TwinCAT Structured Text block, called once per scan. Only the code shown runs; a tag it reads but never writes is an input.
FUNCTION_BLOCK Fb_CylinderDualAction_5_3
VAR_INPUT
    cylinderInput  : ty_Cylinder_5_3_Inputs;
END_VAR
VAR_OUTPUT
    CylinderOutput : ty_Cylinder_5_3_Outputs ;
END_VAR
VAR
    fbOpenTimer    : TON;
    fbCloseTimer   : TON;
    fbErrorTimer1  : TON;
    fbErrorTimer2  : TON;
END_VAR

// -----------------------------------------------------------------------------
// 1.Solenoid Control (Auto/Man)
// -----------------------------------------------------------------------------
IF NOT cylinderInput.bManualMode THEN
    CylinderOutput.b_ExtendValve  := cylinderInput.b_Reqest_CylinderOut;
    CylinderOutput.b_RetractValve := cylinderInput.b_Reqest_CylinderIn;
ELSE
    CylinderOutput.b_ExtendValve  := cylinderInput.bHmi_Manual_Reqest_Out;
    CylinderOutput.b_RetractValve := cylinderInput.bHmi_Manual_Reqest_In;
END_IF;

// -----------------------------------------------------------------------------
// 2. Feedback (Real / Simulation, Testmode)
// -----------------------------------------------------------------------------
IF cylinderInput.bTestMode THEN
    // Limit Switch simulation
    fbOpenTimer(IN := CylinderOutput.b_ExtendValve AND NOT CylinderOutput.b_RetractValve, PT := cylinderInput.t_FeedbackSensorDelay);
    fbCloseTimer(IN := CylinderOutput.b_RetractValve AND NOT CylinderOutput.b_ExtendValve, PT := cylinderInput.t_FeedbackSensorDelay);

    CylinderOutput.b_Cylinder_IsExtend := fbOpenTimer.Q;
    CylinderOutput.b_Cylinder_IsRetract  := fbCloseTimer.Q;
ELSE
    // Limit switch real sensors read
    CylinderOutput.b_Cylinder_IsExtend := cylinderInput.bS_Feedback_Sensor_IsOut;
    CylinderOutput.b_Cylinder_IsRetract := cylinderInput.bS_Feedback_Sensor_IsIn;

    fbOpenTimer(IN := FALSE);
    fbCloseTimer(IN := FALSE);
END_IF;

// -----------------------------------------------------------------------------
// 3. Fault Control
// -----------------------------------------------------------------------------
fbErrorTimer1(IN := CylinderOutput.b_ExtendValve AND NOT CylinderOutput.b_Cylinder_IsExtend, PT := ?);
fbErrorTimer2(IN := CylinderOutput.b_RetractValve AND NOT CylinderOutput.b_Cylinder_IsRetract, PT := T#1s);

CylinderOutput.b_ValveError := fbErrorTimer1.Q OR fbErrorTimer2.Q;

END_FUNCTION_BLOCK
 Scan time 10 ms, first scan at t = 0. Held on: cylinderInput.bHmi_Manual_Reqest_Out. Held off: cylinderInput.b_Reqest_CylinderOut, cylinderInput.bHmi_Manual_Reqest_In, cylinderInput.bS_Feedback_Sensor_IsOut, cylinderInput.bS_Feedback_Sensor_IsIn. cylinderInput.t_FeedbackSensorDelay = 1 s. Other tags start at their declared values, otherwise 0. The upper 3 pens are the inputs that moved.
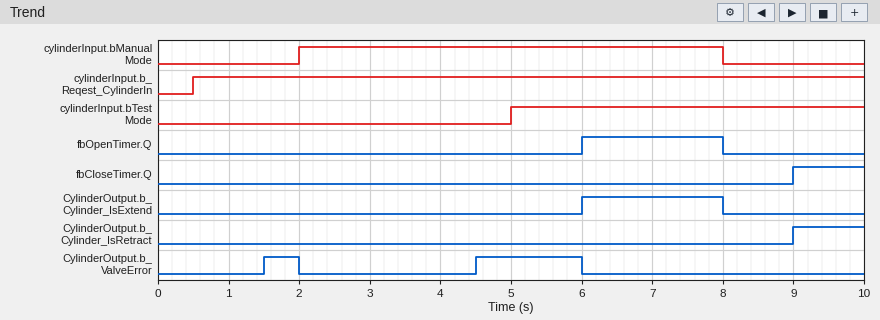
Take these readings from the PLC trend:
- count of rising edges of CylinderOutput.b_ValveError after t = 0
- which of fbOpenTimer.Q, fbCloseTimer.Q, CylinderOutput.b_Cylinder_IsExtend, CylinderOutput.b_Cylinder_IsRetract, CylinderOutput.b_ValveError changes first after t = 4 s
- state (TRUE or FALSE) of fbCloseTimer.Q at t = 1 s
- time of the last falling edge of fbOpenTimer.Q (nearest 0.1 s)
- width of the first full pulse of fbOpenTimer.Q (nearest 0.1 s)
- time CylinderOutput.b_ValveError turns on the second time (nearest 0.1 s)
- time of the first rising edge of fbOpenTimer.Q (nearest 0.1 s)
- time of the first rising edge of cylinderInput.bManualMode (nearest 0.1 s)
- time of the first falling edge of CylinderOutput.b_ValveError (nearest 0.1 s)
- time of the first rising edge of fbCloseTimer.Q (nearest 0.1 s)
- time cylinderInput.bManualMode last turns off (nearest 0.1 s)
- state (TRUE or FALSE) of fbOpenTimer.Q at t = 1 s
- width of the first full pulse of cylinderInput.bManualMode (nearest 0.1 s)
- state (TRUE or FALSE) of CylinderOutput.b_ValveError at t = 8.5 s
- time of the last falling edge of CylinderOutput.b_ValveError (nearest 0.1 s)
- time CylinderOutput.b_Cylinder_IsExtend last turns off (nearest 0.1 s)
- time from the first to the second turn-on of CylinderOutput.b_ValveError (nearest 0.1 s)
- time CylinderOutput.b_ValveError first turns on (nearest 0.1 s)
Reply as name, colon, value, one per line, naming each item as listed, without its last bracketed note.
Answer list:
count of rising edges of CylinderOutput.b_ValveError after t = 0: 2
which of fbOpenTimer.Q, fbCloseTimer.Q, CylinderOutput.b_Cylinder_IsExtend, CylinderOutput.b_Cylinder_IsRetract, CylinderOutput.b_ValveError changes first after t = 4 s: CylinderOutput.b_ValveError
state (TRUE or FALSE) of fbCloseTimer.Q at t = 1 s: FALSE
time of the last falling edge of fbOpenTimer.Q: 8.0 s
width of the first full pulse of fbOpenTimer.Q: 2.0 s
time CylinderOutput.b_ValveError turns on the second time: 4.5 s
time of the first rising edge of fbOpenTimer.Q: 6.0 s
time of the first rising edge of cylinderInput.bManualMode: 2.0 s
time of the first falling edge of CylinderOutput.b_ValveError: 2.0 s
time of the first rising edge of fbCloseTimer.Q: 9.0 s
time cylinderInput.bManualMode last turns off: 8.0 s
state (TRUE or FALSE) of fbOpenTimer.Q at t = 1 s: FALSE
width of the first full pulse of cylinderInput.bManualMode: 6.0 s
state (TRUE or FALSE) of CylinderOutput.b_ValveError at t = 8.5 s: FALSE
time of the last falling edge of CylinderOutput.b_ValveError: 6.0 s
time CylinderOutput.b_Cylinder_IsExtend last turns off: 8.0 s
time from the first to the second turn-on of CylinderOutput.b_ValveError: 3.0 s
time CylinderOutput.b_ValveError first turns on: 1.5 s
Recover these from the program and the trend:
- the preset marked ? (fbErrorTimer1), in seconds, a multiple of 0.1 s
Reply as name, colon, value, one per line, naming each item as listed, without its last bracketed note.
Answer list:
the preset marked ? (fbErrorTimer1), in seconds, a multiple of 0.1 s: 2.5 s
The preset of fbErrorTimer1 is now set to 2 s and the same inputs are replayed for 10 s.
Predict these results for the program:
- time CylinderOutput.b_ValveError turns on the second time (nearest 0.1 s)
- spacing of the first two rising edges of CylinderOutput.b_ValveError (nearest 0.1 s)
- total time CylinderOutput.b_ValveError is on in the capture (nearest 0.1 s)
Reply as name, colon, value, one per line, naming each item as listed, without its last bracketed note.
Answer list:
time CylinderOutput.b_ValveError turns on the second time: 4.0 s
spacing of the first two rising edges of CylinderOutput.b_ValveError: 2.5 s
total time CylinderOutput.b_ValveError is on in the capture: 2.5 s
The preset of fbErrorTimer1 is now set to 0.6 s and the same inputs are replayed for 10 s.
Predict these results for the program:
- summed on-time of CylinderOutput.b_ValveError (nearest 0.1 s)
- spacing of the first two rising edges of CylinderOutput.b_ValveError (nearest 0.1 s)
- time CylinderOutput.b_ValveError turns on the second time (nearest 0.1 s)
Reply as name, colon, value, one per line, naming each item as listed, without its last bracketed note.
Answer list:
summed on-time of CylinderOutput.b_ValveError: 3.9 s
spacing of the first two rising edges of CylinderOutput.b_ValveError: 1.1 s
time CylinderOutput.b_ValveError turns on the second time: 2.6 s
